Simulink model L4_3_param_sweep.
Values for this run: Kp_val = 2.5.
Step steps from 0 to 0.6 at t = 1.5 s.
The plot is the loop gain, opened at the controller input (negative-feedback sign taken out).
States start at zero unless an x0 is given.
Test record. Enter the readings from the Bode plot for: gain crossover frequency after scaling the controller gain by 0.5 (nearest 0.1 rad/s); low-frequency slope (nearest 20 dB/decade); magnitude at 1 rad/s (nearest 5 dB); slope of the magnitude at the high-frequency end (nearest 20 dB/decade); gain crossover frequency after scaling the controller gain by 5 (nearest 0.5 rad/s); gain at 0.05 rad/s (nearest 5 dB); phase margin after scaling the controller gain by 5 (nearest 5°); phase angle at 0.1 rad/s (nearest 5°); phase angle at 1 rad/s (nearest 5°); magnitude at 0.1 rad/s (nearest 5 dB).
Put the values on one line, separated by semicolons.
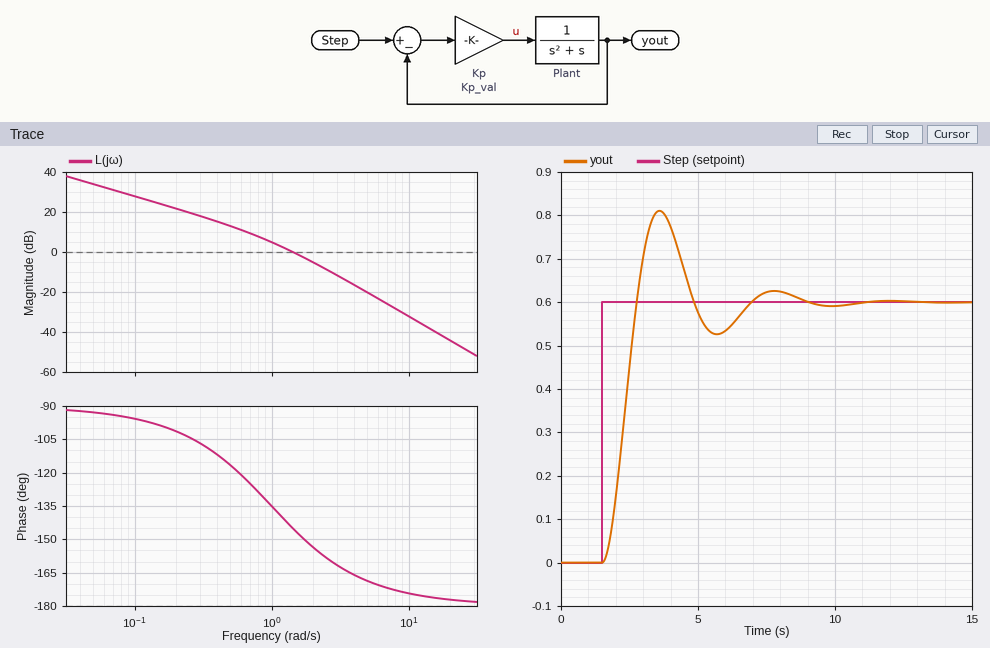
0.9 rad/s; -20 dB/decade; 5 dB; -40 dB/decade; 3.5 rad/s; 35 dB; 15°; -95°; -135°; 30 dB
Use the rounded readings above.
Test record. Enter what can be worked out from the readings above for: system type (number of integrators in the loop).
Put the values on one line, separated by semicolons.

1
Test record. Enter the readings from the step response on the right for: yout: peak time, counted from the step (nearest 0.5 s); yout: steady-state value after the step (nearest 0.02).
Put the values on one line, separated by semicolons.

2.0 s; 0.60
